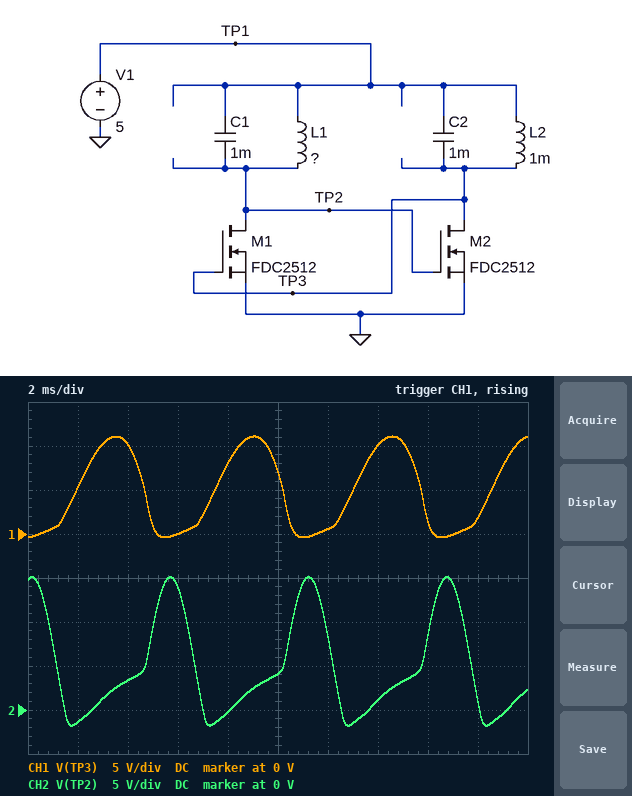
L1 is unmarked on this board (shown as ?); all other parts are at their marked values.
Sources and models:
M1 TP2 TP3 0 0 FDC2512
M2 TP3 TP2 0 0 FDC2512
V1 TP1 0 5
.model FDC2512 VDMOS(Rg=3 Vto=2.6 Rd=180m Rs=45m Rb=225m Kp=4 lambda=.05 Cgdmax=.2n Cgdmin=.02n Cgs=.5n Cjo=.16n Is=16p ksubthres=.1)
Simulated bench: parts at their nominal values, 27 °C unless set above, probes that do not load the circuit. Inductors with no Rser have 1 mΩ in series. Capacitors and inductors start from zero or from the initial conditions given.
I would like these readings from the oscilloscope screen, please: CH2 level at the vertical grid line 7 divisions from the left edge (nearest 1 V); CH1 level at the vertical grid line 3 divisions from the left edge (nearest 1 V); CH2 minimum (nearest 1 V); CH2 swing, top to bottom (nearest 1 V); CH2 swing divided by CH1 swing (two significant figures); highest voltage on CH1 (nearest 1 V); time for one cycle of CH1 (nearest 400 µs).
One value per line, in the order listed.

1 V
0 V
-2 V
17 V
1.5
11 V
5.6 ms
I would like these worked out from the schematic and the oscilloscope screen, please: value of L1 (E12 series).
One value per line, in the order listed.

390 µH
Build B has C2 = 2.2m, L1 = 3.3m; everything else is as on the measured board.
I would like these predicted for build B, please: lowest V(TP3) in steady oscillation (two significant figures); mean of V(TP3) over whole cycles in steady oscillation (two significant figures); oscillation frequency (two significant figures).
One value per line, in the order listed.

-1.4 V
5.0 V
85 Hz
